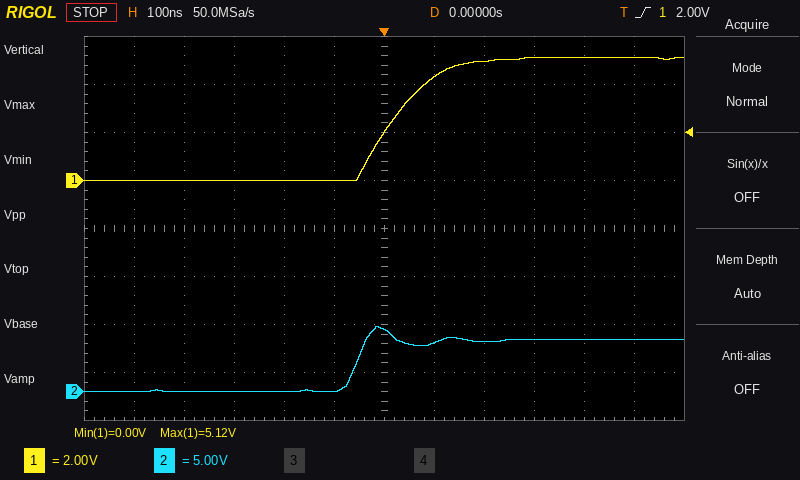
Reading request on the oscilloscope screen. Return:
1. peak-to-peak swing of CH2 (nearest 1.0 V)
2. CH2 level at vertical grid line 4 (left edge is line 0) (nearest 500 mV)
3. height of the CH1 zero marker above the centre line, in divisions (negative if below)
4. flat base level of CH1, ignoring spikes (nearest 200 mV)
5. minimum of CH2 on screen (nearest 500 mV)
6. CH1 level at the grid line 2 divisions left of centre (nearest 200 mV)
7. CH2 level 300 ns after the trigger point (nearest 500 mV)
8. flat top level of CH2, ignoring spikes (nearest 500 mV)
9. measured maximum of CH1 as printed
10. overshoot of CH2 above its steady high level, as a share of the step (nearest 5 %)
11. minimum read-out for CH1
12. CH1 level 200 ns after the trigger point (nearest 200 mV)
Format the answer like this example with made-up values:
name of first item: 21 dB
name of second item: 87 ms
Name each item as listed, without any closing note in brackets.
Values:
peak-to-peak swing of CH2: 7.0 V
CH2 level at vertical grid line 4 (left edge is line 0): 0.0 V
height of the CH1 zero marker above the centre line, in divisions: +1.0 div
flat base level of CH1, ignoring spikes: 0.0 V
minimum of CH2 on screen: 0.0 V
CH1 level at the grid line 2 divisions left of centre: 0.0 V
CH2 level 300 ns after the trigger point: 5.5 V
flat top level of CH2, ignoring spikes: 5.5 V
measured maximum of CH1 as printed: 5.12 V
overshoot of CH2 above its steady high level, as a share of the step: 25 %
minimum read-out for CH1: 0.00 V
CH1 level 200 ns after the trigger point: 5.0 V
